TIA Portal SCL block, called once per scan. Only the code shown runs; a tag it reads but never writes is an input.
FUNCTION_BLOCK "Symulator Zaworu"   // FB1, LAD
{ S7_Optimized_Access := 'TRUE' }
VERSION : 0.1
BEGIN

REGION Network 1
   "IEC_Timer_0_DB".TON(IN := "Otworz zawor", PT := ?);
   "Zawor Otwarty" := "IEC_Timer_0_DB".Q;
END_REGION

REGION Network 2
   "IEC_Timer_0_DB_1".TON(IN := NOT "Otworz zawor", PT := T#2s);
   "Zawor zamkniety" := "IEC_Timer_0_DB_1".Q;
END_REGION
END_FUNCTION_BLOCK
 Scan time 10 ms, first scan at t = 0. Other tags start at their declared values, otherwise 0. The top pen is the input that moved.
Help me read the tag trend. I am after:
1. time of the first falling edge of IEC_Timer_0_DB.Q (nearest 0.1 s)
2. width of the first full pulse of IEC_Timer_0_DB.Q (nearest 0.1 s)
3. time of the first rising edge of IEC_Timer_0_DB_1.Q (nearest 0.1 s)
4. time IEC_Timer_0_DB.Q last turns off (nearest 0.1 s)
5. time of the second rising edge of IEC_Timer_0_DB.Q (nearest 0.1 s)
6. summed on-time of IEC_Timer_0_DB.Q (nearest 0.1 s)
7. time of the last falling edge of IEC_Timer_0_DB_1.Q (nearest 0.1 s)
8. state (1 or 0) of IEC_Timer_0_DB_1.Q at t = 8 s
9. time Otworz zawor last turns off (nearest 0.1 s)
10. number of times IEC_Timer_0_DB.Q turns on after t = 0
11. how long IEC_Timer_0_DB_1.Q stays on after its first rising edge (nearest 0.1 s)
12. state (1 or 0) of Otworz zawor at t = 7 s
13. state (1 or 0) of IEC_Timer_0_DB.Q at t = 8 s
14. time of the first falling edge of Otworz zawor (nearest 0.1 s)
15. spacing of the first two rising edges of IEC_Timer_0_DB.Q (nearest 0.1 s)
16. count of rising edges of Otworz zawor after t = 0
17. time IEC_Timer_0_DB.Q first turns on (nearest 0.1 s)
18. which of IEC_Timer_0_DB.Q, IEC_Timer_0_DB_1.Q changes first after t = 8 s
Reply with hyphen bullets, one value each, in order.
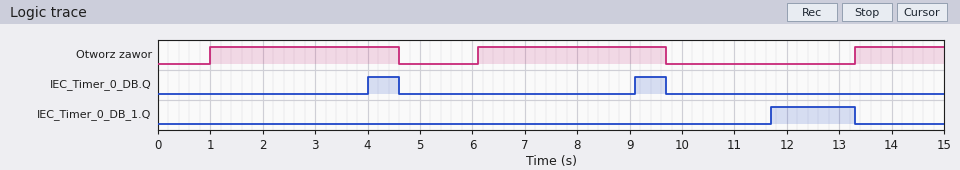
- 4.6 s
- 0.6 s
- 11.7 s
- 9.7 s
- 9.1 s
- 1.2 s
- 13.3 s
- 0
- 9.7 s
- 2
- 1.6 s
- 1
- 0
- 4.6 s
- 5.1 s
- 3
- 4.0 s
- IEC_Timer_0_DB.Q
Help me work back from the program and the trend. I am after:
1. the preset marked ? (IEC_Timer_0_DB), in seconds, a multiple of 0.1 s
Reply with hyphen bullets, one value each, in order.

- 3.0 s
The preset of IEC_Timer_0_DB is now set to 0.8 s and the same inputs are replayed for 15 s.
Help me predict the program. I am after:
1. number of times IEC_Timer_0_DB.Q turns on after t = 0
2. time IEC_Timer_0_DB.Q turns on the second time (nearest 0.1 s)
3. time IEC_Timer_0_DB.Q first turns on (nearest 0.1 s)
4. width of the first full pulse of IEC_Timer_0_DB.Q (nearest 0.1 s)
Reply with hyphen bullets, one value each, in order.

- 3
- 6.9 s
- 1.8 s
- 2.8 s
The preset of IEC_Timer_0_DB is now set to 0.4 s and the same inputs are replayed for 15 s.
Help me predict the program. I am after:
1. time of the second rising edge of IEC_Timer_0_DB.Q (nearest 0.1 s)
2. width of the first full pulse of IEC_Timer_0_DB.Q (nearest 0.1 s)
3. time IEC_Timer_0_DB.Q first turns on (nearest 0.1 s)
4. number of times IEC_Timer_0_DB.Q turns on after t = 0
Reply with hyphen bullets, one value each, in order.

- 6.5 s
- 3.2 s
- 1.4 s
- 3
